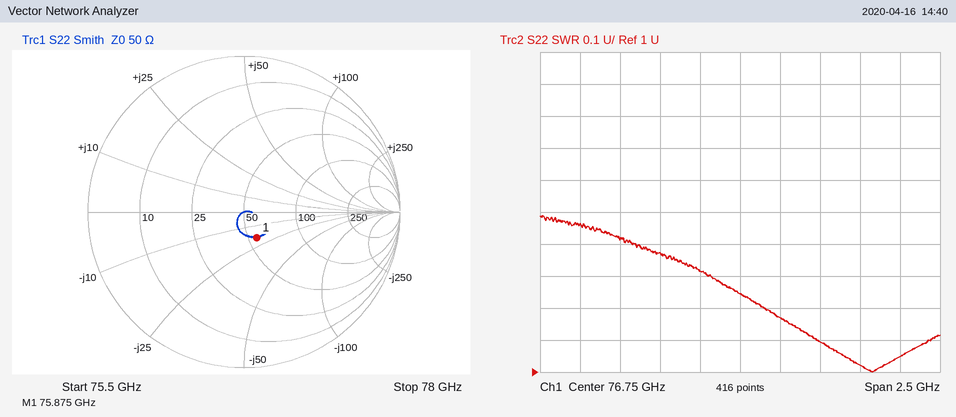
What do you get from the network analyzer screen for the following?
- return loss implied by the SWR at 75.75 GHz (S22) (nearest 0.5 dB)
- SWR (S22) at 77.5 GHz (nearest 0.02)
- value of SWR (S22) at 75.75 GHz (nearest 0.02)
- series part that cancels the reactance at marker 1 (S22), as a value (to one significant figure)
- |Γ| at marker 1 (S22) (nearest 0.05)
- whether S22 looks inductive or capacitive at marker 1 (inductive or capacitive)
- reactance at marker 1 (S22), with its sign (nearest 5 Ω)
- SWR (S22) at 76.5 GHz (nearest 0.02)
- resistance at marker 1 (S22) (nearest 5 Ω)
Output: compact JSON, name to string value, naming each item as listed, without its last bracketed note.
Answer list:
{"return loss implied by the SWR at 75.75 GHz (S22)": "14.5 dB", "SWR (S22) at 77.5 GHz": "1.02", "value of SWR (S22) at 75.75 GHz": "1.46", "series part that cancels the reactance at marker 1 (S22), as a value": "40 pH", "|Γ| at marker 1 (S22)": "0.20", "whether S22 looks inductive or capacitive at marker 1": "capacitive", "reactance at marker 1 (S22), with its sign": "-20 Ω", "SWR (S22) at 76.5 GHz": "1.32", "resistance at marker 1 (S22)": "55 Ω"}
